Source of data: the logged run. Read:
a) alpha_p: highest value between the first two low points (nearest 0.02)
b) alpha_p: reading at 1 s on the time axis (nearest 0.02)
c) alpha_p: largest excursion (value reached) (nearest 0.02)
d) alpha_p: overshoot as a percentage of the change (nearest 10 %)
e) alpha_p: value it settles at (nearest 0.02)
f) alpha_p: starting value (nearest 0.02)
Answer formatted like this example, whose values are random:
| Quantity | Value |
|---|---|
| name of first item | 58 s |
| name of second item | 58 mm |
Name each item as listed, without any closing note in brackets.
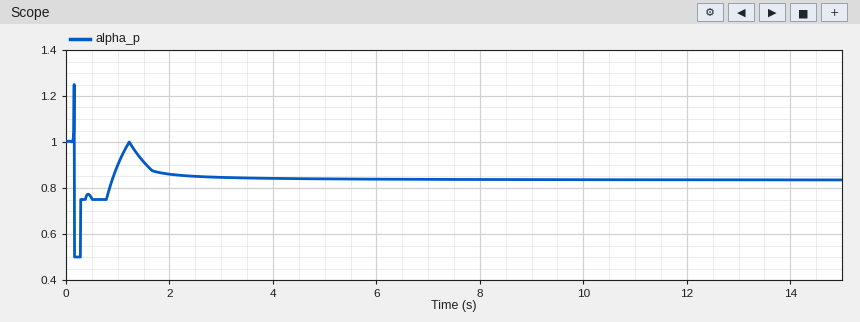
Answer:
| Quantity | Value |
|---|---|
| alpha_p: highest value between the first two low points | 0.78 |
| alpha_p: reading at 1 s on the time axis | 0.90 |
| alpha_p: largest excursion (value reached) | 0.50 |
| alpha_p: overshoot as a percentage of the change | 200 % |
| alpha_p: value it settles at | 0.84 |
| alpha_p: starting value | 1.00 |
